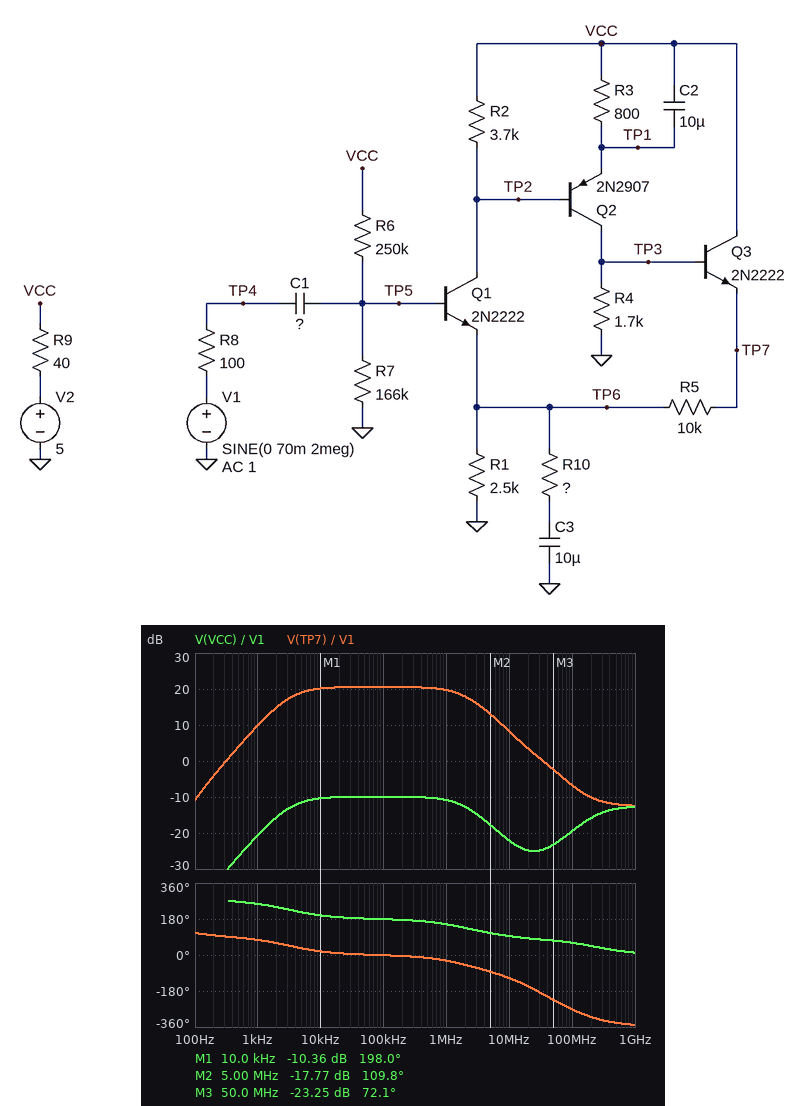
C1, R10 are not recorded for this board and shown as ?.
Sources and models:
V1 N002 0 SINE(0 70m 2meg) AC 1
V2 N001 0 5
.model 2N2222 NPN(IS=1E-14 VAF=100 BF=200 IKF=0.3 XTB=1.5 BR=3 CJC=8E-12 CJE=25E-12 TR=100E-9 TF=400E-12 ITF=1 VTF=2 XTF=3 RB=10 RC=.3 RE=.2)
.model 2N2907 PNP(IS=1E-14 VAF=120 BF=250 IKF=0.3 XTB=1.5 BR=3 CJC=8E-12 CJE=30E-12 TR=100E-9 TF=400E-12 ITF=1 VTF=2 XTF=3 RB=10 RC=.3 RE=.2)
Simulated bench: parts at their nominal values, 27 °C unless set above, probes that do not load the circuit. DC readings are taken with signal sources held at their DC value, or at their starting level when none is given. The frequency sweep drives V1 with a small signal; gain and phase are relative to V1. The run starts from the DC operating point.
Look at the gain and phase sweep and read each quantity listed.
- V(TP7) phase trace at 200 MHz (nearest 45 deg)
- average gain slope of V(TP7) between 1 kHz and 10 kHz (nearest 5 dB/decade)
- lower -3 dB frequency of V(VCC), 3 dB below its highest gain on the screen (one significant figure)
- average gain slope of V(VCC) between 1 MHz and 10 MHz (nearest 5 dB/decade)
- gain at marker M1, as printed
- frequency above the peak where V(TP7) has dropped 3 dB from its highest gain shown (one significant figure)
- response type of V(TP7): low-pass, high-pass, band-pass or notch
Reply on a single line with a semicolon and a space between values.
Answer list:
-315 deg; 10 dB/decade; 3 kHz; -10 dB/decade; -10.36 dB; 2 MHz; band-pass
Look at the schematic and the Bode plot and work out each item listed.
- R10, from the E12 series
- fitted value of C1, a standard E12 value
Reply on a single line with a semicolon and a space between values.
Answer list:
1.5 kΩ; 560 pF
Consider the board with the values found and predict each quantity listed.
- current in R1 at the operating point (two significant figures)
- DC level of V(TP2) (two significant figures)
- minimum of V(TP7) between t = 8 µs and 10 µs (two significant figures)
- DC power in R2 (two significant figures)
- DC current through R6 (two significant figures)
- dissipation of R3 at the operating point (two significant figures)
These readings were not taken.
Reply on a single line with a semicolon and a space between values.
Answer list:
450 µA; 3.4 V; 820 mV; 660 µW; 13 µA; 1.0 mW
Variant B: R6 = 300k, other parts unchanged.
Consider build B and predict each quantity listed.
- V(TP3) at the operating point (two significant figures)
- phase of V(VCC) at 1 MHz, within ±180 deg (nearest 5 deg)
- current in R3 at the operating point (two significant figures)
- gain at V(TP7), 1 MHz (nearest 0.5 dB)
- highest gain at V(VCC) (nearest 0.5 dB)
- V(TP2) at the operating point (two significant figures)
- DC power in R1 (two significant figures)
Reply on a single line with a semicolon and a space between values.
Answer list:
1.5 V; 145 deg; 880 µA; 19.0 dB; -7.5 dB; 3.6 V; 350 µW
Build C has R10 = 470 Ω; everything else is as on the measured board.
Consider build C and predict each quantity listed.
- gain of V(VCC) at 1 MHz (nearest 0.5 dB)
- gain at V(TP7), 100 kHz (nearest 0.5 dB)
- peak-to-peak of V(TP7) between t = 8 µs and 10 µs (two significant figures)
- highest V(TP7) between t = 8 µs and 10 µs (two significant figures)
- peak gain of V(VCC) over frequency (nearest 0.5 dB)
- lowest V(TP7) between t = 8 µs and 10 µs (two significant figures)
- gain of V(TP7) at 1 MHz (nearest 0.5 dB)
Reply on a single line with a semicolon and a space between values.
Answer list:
-4.0 dB; 27.5 dB; 2.1 V; 2.4 V; -3.0 dB; 300 mV; 26.5 dB
